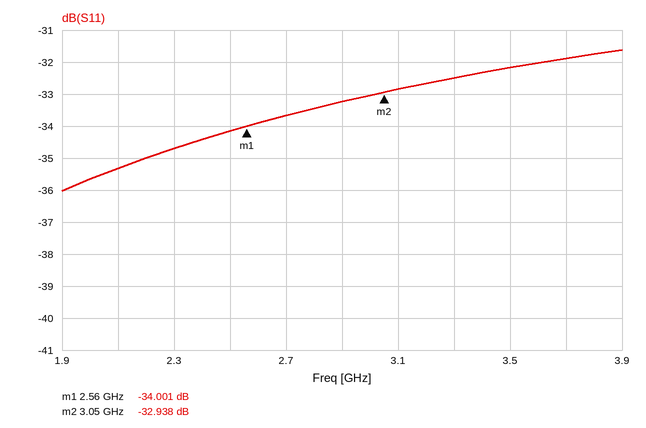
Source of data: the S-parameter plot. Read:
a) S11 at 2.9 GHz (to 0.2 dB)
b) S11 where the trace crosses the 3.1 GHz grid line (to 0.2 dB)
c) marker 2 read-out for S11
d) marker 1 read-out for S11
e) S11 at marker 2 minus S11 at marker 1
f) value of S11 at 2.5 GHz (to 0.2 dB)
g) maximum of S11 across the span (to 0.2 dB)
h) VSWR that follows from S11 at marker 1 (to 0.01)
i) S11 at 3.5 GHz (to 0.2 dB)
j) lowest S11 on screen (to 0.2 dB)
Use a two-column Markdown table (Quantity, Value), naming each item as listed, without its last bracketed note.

| Quantity | Value |
|---|---|
| S11 at 2.9 GHz | -33.2 dB |
| S11 where the trace crosses the 3.1 GHz grid line | -32.8 dB |
| marker 2 read-out for S11 | -32.938 dB |
| marker 1 read-out for S11 | -34.001 dB |
| S11 at marker 2 minus S11 at marker 1 | 1.063 dB |
| value of S11 at 2.5 GHz | -34.2 dB |
| maximum of S11 across the span | -31.6 dB |
| VSWR that follows from S11 at marker 1 | 1.04 |
| S11 at 3.5 GHz | -32.2 dB |
| lowest S11 on screen | -36.0 dB |
